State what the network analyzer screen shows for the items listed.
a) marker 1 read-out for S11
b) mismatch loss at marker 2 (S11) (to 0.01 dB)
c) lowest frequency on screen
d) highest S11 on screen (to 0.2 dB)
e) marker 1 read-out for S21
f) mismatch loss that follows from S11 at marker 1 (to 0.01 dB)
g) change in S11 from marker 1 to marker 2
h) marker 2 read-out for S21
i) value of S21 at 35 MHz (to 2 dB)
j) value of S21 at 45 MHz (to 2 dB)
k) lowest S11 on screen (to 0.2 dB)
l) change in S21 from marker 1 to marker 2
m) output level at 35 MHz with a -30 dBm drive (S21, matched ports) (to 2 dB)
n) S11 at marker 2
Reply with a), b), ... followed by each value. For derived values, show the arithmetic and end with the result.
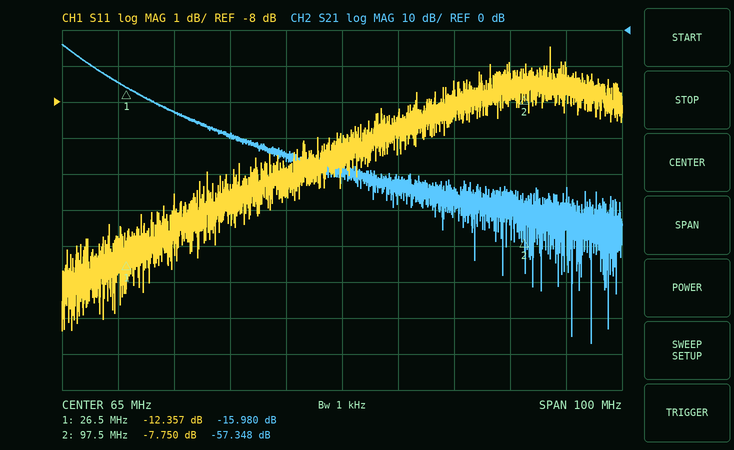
a) -12.357 dB
b) −10 log10(1 − 10^(-7.75/10)) ≈ 0.80 dB
c) 15 MHz
d) -6.4 dB
e) -15.980 dB
f) −10 log10(1 − 10^(-12.357/10)) ≈ 0.26 dB
g) -7.75 − (-12.357) = 4.607 dB
h) -57.348 dB
i) -22 dB
j) -30 dB
k) -14.4 dB
l) -57.348 − (-15.98) = -41.368 dB
m) -30 dBm + (-22 dB) = -52 dBm
n) -7.750 dB
